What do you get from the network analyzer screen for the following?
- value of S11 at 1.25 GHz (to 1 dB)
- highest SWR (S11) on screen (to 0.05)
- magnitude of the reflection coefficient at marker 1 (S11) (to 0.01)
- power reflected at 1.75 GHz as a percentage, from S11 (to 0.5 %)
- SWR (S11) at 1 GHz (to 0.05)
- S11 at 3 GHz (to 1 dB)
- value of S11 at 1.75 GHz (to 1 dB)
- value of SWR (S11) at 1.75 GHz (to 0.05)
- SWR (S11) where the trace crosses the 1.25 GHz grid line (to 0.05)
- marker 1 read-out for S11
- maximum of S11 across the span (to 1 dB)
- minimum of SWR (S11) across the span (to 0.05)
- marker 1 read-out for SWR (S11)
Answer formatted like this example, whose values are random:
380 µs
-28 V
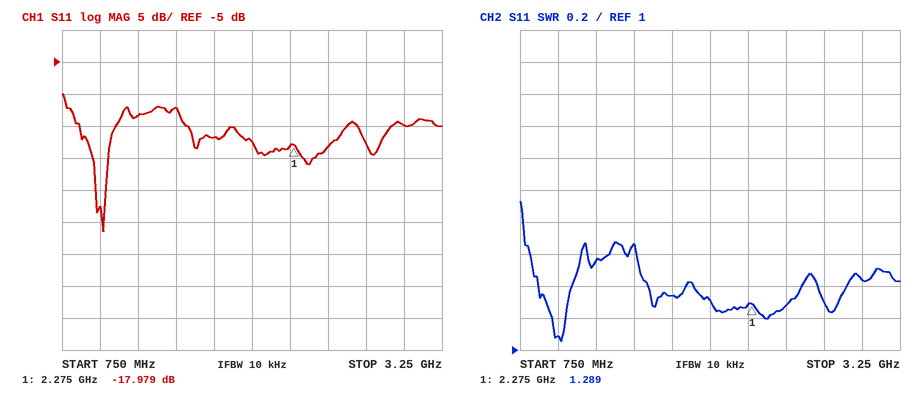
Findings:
-13 dB
1.95
0.13
2.0 %
1.10
-15 dB
-17 dB
1.35
1.55
-17.979 dB
-10 dB
1.05
1.289
